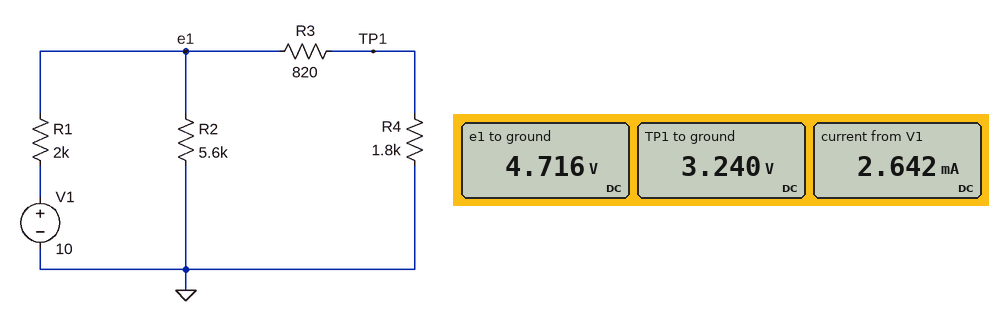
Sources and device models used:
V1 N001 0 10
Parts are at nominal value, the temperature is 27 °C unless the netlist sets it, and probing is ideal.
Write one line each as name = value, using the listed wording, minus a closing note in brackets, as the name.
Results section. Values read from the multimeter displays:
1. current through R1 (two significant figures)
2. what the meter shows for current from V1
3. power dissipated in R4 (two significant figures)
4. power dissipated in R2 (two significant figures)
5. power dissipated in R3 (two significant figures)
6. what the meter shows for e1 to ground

current through R1 = 2.6 mA
what the meter shows for current from V1 = 2.642 mA
power dissipated in R4 = 5.8 mW
power dissipated in R2 = 4.0 mW
power dissipated in R3 = 2.7 mW
what the meter shows for e1 to ground = 4.716 V
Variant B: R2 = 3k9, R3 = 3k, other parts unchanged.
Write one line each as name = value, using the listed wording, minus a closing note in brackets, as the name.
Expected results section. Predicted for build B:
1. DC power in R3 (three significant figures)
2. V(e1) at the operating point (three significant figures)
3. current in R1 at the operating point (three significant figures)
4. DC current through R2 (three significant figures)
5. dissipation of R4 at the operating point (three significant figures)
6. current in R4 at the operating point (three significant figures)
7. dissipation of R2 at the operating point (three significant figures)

DC power in R3 = 3.50 mW
V(e1) at the operating point = 5.18 V
current in R1 at the operating point = 2.41 mA
DC current through R2 = 1.33 mA
dissipation of R4 at the operating point = 2.10 mW
current in R4 at the operating point = 1.08 mA
dissipation of R2 at the operating point = 6.89 mW
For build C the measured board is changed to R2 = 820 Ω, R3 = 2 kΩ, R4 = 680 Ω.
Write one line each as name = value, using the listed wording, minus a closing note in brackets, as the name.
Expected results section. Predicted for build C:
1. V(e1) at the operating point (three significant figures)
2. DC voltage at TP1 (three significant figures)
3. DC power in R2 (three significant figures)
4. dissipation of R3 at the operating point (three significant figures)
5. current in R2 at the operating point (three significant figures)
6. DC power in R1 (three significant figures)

V(e1) at the operating point = 2.39 V
DC voltage at TP1 = 606 mV
DC power in R2 = 6.96 mW
dissipation of R3 at the operating point = 1.59 mW
current in R2 at the operating point = 2.91 mA
DC power in R1 = 29.0 mW
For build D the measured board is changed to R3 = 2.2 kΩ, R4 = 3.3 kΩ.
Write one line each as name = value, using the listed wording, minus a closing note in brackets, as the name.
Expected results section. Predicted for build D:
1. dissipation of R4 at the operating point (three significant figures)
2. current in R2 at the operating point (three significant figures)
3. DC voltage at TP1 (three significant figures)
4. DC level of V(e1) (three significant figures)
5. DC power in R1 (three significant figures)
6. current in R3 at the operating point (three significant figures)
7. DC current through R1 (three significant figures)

dissipation of R4 at the operating point = 3.68 mW
current in R2 at the operating point = 1.04 mA
DC voltage at TP1 = 3.49 V
DC level of V(e1) = 5.81 V
DC power in R1 = 8.77 mW
current in R3 at the operating point = 1.06 mA
DC current through R1 = 2.09 mA
